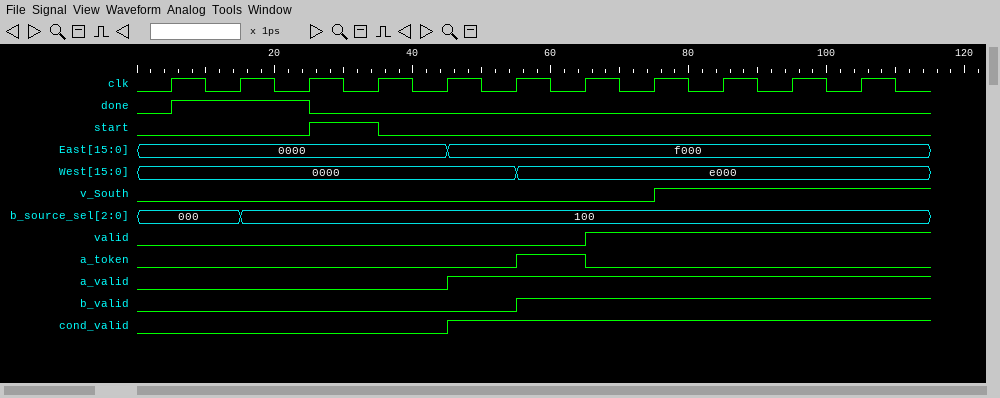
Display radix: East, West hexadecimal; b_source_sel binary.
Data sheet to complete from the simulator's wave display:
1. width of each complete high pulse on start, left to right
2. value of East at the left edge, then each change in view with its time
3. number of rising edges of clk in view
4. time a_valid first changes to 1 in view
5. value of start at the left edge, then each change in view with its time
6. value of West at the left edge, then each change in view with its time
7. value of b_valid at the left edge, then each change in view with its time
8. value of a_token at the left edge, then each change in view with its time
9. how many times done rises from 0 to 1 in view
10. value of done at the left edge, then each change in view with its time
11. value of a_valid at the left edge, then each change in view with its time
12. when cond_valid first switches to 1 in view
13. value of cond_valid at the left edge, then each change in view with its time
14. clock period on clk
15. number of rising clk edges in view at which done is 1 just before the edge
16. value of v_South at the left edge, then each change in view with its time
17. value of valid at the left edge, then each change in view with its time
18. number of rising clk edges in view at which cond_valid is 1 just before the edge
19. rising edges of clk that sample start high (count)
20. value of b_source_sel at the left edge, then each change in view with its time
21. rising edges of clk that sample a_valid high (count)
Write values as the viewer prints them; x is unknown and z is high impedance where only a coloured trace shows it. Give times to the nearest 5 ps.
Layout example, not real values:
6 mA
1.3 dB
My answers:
10 ps
0000, f000 at 45 ps
11
45 ps
0, 1 at 25 ps, 0 at 35 ps
0000, e000 at 55 ps
0, 1 at 55 ps
0, 1 at 55 ps, 0 at 65 ps
1
0, 1 at 5 ps, 0 at 25 ps
0, 1 at 45 ps
45 ps
0, 1 at 45 ps
10 ps
2
0, 1 at 75 ps
0, 1 at 65 ps
6
1
000, 100 at 15 ps
6
